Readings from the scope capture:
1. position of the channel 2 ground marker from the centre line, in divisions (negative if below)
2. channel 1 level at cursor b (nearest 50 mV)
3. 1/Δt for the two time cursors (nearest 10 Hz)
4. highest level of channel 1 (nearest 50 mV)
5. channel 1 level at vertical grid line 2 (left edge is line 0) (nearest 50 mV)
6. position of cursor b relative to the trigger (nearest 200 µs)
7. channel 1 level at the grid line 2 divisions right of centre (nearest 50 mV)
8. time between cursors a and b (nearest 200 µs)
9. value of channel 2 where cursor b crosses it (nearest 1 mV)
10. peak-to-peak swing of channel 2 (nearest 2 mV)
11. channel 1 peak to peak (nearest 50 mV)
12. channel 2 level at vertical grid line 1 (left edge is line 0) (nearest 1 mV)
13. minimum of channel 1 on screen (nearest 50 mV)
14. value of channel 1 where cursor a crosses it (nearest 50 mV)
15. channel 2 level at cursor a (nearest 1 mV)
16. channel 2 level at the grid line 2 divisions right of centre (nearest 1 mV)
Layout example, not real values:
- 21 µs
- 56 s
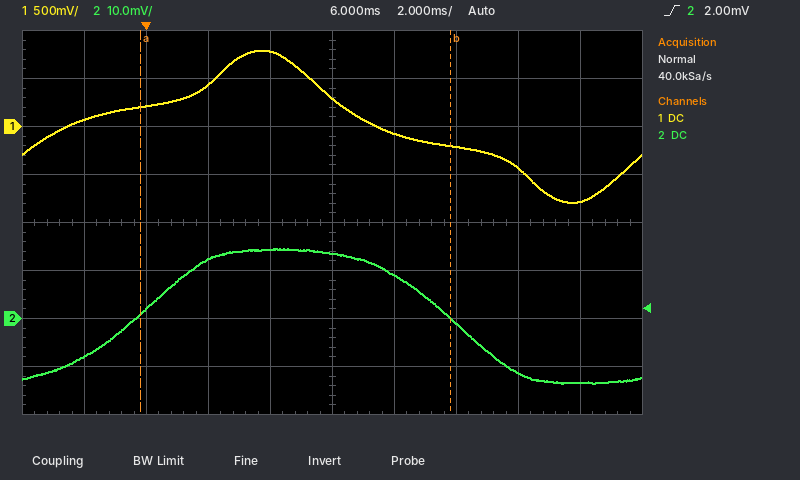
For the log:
- -2.0 div
- -200 mV
- 100 Hz
- 800 mV
- 200 mV
- +9.8 ms
- -200 mV
- 10.0 ms
- 0 mV
- 28 mV
- 1.60 V
- -8 mV
- -800 mV
- 200 mV
- 1 mV
- -1 mV
